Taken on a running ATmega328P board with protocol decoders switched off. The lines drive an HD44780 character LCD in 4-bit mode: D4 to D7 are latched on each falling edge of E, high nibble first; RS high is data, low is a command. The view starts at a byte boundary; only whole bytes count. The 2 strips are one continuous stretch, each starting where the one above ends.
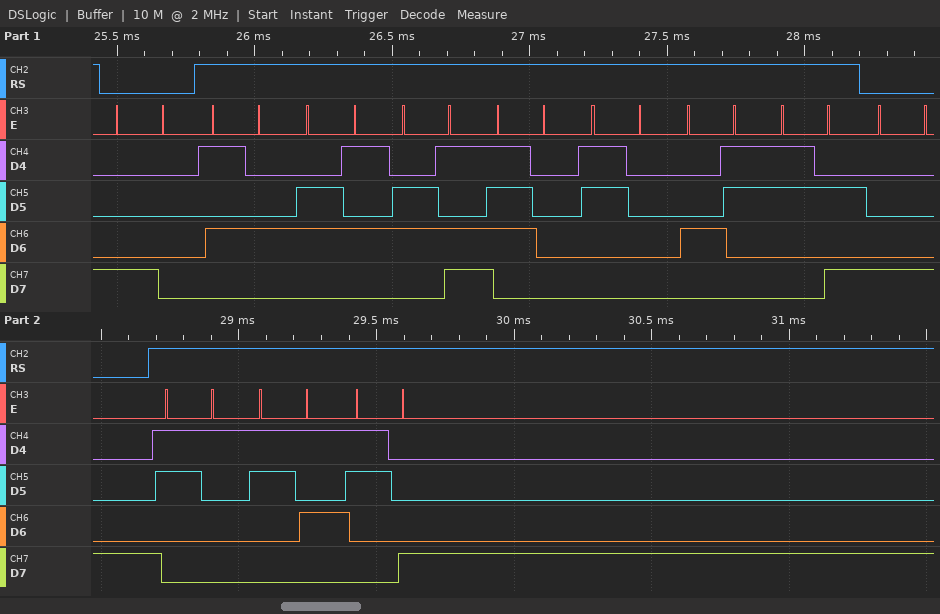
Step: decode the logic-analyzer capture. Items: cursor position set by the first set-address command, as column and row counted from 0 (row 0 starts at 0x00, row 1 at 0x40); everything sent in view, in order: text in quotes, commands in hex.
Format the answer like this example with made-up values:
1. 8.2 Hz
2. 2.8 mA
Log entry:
1. column 0, row 0
2. 0x80 "Temp0C:" 0x88 "158"
